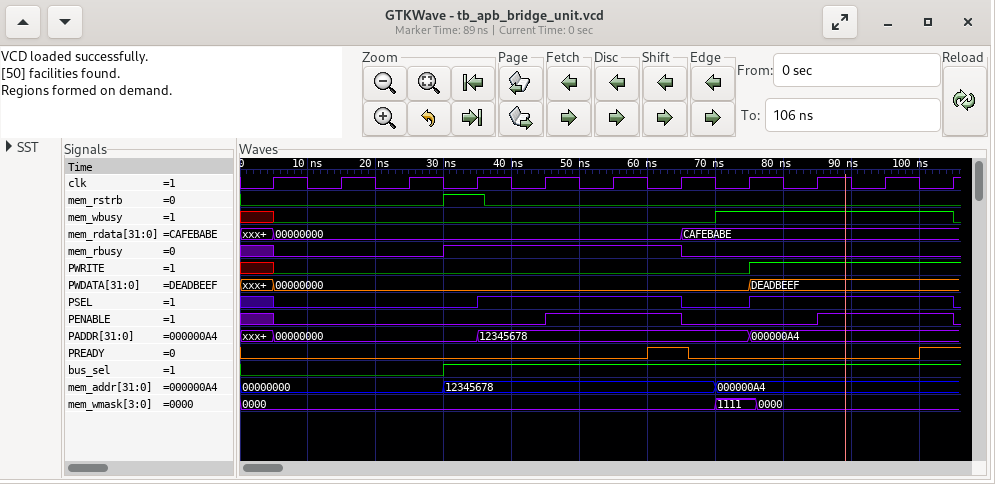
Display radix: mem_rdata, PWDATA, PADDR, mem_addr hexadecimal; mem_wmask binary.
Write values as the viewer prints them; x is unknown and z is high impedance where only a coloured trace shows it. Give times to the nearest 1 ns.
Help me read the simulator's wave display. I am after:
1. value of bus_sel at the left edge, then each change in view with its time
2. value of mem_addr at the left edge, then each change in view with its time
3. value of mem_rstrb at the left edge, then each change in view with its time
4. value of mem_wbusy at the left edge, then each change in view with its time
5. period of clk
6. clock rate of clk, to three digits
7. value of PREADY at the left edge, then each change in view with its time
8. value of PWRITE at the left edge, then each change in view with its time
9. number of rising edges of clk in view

0, 1 at 30 ns
00000000, 12345678 at 30 ns, 000000A4 at 70 ns
0, 1 at 30 ns, 0 at 36 ns
x, 0 at 5 ns, 1 at 70 ns, 0 at 105 ns
10 ns
100 MHz
0, 1 at 60 ns, 0 at 66 ns, 1 at 100 ns
x, 0 at 5 ns, 1 at 75 ns
11
